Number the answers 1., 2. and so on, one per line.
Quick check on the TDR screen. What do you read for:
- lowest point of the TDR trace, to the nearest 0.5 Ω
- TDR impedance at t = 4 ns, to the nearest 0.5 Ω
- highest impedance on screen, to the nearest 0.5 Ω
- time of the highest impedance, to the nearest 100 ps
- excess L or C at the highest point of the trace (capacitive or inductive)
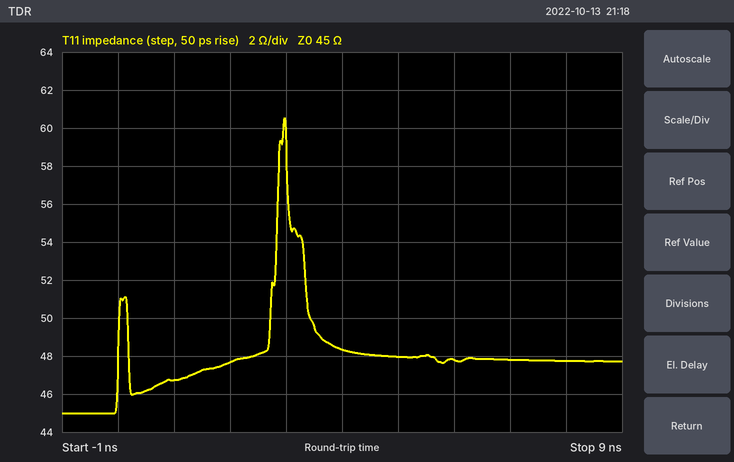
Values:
1. 45.0 Ω
2. 48.5 Ω
3. 60.5 Ω
4. 3.0 ns
5. inductive
